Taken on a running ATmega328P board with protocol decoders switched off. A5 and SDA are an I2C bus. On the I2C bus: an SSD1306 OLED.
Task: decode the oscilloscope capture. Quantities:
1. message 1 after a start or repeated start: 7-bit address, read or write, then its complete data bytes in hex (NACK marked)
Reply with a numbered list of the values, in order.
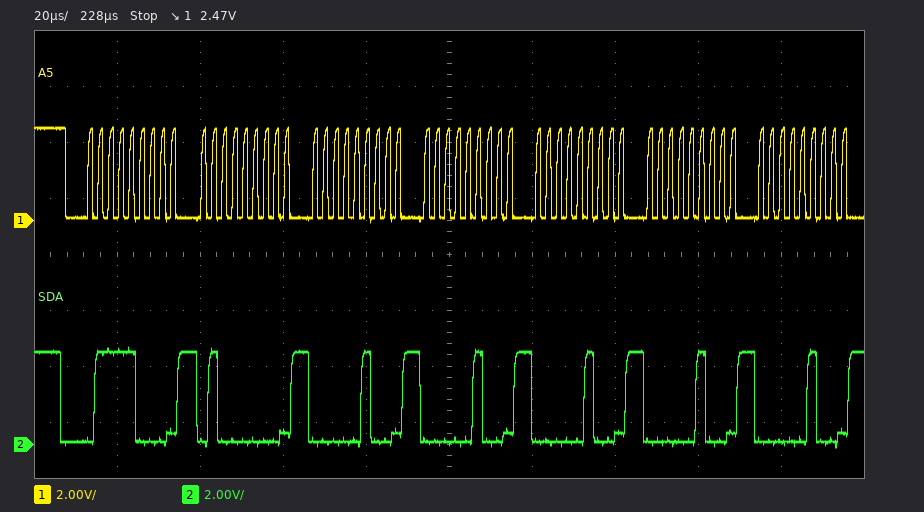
1. 0x3C write: 40 04 04 04 04 04
